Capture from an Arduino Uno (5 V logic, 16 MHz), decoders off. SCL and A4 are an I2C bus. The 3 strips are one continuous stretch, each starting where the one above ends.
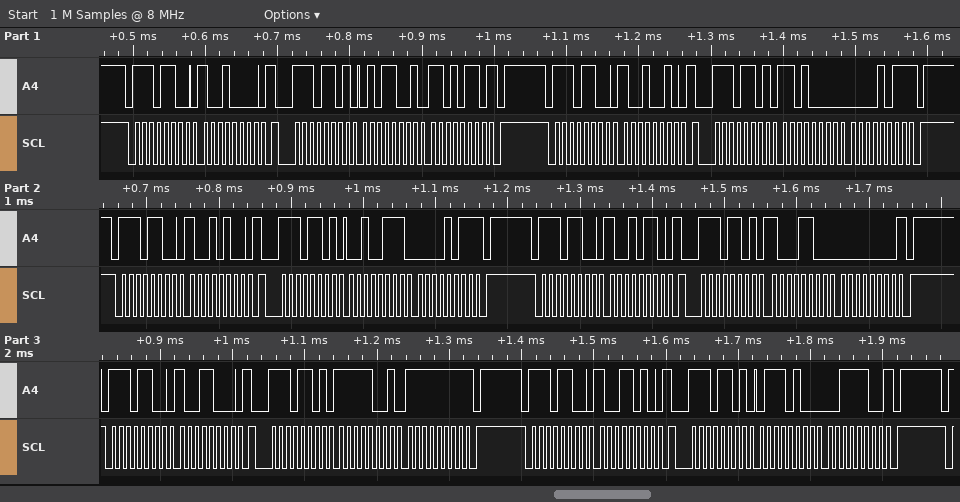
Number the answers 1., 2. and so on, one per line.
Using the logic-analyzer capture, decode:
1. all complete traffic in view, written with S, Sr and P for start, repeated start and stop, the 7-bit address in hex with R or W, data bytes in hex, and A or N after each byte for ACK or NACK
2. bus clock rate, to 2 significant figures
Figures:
1. S 76W A 90 A Sr 76R A 59 A D6 N P S 76W A 92 A Sr 76R A D0 A 0B N P S 76W A 94 A Sr 76R A 27 A 0B N P S 76W A 96 A Sr 76R A 8C A 00 N P S 76W A 98 A Sr 76R A F9 A FF N P S 76W A 9A A Sr 76R A 74 A 3C N P
2. 100 kHz
